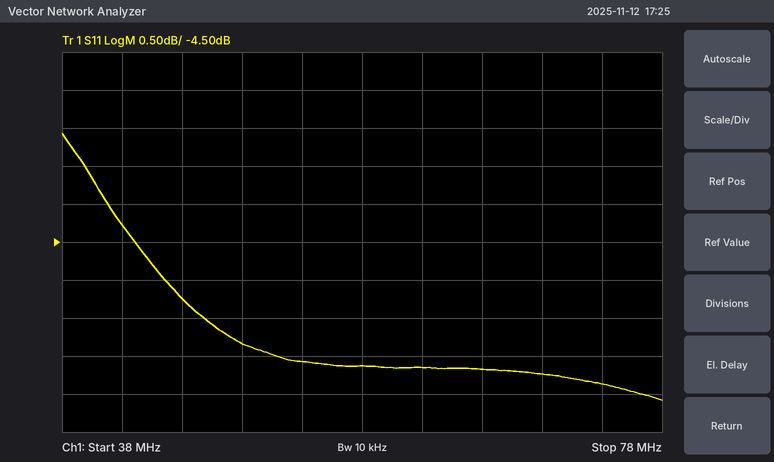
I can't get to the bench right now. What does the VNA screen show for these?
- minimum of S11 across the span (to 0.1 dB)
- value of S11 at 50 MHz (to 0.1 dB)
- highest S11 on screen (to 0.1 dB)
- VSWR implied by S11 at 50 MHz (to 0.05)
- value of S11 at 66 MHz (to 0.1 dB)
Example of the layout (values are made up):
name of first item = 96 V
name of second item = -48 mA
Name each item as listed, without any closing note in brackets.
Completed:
minimum of S11 across the span = -6.6 dB
value of S11 at 50 MHz = -5.8 dB
highest S11 on screen = -3.1 dB
VSWR implied by S11 at 50 MHz = 3.10
value of S11 at 66 MHz = -6.2 dB
